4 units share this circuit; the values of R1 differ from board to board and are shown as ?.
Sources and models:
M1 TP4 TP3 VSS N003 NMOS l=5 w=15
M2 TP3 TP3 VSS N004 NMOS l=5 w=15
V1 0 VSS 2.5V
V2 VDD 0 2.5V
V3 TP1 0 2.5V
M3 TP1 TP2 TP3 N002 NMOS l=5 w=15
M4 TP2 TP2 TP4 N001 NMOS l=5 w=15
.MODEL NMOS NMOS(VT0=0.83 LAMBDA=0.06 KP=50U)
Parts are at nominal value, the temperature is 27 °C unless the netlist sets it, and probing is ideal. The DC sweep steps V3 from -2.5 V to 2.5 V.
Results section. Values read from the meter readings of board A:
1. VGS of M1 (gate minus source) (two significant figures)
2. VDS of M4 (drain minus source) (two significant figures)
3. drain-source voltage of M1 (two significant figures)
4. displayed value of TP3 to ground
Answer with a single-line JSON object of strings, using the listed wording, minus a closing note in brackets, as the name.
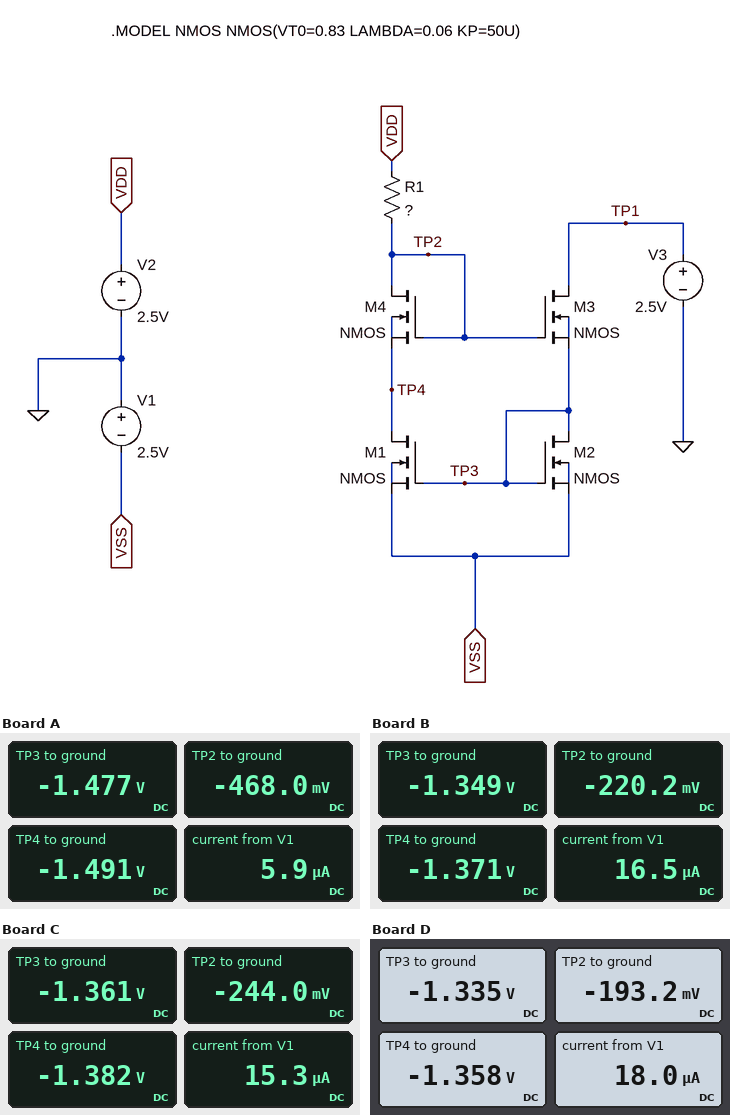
{"VGS of M1 (gate minus source)": "1.0 V", "VDS of M4 (drain minus source)": "1.0 V", "drain-source voltage of M1": "1.0 V", "displayed value of TP3 to ground": "-1.477 V"}
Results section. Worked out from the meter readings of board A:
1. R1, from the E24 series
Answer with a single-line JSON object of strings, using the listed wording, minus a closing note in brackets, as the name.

{"R1, from the E24 series": "1 MΩ"}
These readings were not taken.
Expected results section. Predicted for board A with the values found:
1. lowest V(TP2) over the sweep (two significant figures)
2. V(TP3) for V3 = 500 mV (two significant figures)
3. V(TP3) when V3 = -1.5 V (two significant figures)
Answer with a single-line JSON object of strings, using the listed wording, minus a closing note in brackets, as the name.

{"lowest V(TP2) over the sweep": "-470 mV", "V(TP3) for V3 = 500 mV": "-1.5 V", "V(TP3) when V3 = -1.5 V": "-1.5 V"}
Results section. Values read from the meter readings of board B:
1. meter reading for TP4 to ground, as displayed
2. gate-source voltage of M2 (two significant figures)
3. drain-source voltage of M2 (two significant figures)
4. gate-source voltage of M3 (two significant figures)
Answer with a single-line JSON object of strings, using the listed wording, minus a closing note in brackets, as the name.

{"meter reading for TP4 to ground, as displayed": "-1.371 V", "gate-source voltage of M2": "1.2 V", "drain-source voltage of M2": "1.2 V", "gate-source voltage of M3": "1.1 V"}
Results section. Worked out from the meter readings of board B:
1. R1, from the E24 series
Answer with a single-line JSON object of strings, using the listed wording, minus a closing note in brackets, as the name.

{"R1, from the E24 series": "330 kΩ"}
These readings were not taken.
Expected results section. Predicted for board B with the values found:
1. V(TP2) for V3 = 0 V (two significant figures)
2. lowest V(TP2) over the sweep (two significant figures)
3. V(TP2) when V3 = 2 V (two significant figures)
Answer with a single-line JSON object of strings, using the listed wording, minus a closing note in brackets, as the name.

{"V(TP2) for V3 = 0 V": "-200 mV", "lowest V(TP2) over the sweep": "-220 mV", "V(TP2) when V3 = 2 V": "-220 mV"}
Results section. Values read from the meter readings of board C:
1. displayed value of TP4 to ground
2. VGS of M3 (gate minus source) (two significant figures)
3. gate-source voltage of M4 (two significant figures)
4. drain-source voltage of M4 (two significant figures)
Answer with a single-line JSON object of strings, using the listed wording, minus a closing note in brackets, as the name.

{"displayed value of TP4 to ground": "-1.382 V", "VGS of M3 (gate minus source)": "1.1 V", "gate-source voltage of M4": "1.1 V", "drain-source voltage of M4": "1.1 V"}
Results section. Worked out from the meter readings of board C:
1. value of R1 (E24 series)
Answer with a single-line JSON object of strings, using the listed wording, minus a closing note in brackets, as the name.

{"value of R1": "360 kΩ"}
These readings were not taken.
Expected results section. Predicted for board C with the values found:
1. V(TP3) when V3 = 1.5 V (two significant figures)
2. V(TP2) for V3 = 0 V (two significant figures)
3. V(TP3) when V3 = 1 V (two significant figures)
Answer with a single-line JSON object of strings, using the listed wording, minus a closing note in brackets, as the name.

{"V(TP3) when V3 = 1.5 V": "-1.4 V", "V(TP2) for V3 = 0 V": "-230 mV", "V(TP3) when V3 = 1 V": "-1.4 V"}
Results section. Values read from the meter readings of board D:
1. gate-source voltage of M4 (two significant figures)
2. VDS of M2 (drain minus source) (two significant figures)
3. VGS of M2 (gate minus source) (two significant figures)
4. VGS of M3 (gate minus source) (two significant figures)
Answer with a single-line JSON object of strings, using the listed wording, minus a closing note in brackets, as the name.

{"gate-source voltage of M4": "1.2 V", "VDS of M2 (drain minus source)": "1.2 V", "VGS of M2 (gate minus source)": "1.2 V", "VGS of M3 (gate minus source)": "1.1 V"}
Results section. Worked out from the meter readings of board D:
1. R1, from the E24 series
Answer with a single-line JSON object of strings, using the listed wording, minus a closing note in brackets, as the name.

{"R1, from the E24 series": "300 kΩ"}
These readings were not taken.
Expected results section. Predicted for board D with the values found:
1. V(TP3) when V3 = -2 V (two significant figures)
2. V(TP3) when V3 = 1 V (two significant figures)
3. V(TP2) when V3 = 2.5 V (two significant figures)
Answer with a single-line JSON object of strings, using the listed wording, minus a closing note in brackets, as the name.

{"V(TP3) when V3 = -2 V": "-2.0 V", "V(TP3) when V3 = 1 V": "-1.3 V", "V(TP2) when V3 = 2.5 V": "-190 mV"}
